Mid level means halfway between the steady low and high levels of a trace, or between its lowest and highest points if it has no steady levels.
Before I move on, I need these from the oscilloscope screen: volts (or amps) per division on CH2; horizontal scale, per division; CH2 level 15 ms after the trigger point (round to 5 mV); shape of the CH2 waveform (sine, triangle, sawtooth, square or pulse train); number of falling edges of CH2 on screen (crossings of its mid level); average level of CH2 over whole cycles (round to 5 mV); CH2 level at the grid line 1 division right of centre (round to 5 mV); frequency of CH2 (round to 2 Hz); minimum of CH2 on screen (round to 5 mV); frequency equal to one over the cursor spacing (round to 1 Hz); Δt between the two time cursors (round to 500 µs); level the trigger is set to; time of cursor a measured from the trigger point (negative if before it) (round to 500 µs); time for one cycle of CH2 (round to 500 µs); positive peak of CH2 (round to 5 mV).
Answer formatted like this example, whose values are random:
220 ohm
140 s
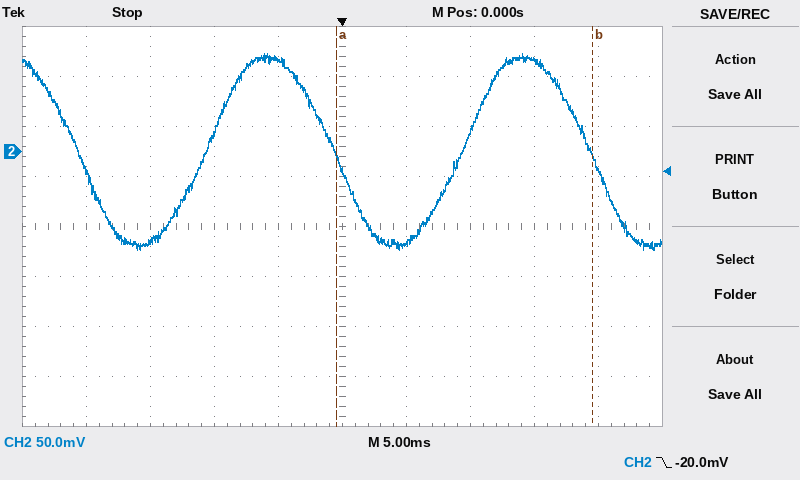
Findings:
50 mV
5 ms
90 mV
sine
3
0 mV
-90 mV
50 Hz
-100 mV
50 Hz
20.0 ms
-20.0 mV
-500 µs
20.0 ms
100 mV
